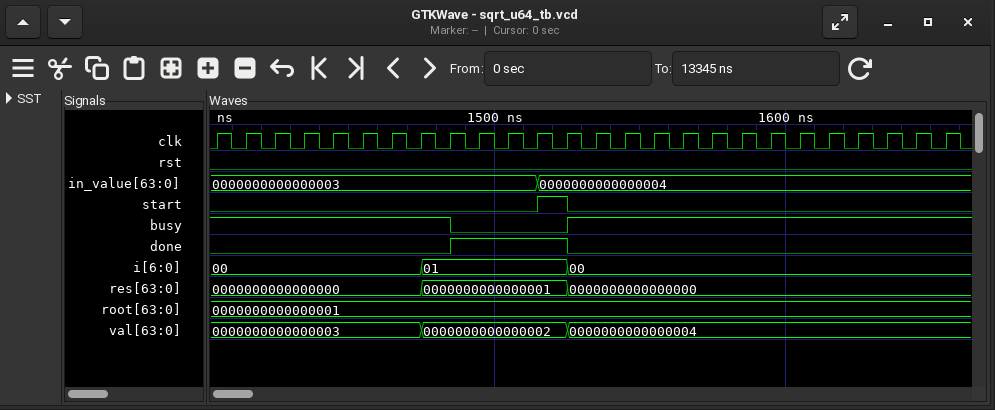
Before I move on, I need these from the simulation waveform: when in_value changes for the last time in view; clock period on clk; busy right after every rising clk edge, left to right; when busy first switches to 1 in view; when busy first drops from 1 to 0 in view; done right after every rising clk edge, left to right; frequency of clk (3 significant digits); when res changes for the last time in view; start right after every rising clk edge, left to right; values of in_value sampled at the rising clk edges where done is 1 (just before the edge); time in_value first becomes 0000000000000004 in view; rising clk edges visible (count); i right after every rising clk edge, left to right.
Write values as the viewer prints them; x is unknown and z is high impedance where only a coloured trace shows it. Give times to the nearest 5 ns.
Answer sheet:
1515 ns
10 ns
1 1 1 1 1 1 1 1 0 0 0 0 1 1 1 1 1 1 1 1 1 1 1 1 1 1
1525 ns
1485 ns
0 0 0 0 0 0 0 0 1 1 1 1 0 0 0 0 0 0 0 0 0 0 0 0 0 0
100 MHz
1525 ns
0 0 0 0 0 0 0 0 0 0 0 1 0 0 0 0 0 0 0 0 0 0 0 0 0 0
0000000000000003, 0000000000000003, 0000000000000003, 0000000000000004
1515 ns
26
00, 00, 00, 00, 00, 00, 00, 01, 01, 01, 01, 01, 00, 00, 00, 00, 00, 00, 00, 00, 00, 00, 00, 00, 00, 00
